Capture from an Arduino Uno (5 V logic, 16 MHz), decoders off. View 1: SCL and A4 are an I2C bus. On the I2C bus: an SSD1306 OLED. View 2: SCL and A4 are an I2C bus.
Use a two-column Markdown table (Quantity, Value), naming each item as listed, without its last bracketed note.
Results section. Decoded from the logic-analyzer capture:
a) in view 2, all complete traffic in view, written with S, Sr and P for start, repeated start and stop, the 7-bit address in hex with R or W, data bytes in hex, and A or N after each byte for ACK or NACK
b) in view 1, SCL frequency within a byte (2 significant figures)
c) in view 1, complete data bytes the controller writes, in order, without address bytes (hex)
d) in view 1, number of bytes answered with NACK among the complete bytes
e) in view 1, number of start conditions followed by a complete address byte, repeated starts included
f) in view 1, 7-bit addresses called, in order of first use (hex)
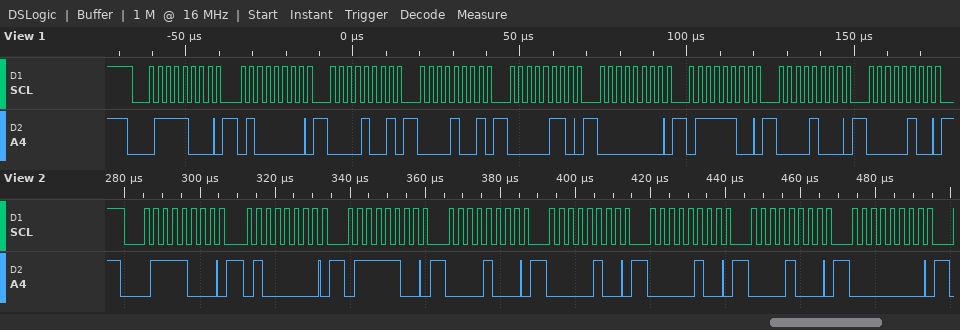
| Quantity | Value |
|---|---|
| in view 2, all complete traffic in view, written with S, Sr and P for start, repeated start and stop, the 7-bit address in hex with R or W, data bytes in hex, and A or N after each byte for ACK or NACK | S 3CW A 40 A 7C A 08 A 04 A 04 A 08 A 00 A |
| in view 1, SCL frequency within a byte | 400 kHz |
| in view 1, complete data bytes the controller writes, in order, without address bytes | 40 09 09 06 00 7C 08 04 |
| in view 1, number of bytes answered with NACK among the complete bytes | 0 |
| in view 1, number of start conditions followed by a complete address byte, repeated starts included | 1 |
| in view 1, 7-bit addresses called, in order of first use | 0x3C |
